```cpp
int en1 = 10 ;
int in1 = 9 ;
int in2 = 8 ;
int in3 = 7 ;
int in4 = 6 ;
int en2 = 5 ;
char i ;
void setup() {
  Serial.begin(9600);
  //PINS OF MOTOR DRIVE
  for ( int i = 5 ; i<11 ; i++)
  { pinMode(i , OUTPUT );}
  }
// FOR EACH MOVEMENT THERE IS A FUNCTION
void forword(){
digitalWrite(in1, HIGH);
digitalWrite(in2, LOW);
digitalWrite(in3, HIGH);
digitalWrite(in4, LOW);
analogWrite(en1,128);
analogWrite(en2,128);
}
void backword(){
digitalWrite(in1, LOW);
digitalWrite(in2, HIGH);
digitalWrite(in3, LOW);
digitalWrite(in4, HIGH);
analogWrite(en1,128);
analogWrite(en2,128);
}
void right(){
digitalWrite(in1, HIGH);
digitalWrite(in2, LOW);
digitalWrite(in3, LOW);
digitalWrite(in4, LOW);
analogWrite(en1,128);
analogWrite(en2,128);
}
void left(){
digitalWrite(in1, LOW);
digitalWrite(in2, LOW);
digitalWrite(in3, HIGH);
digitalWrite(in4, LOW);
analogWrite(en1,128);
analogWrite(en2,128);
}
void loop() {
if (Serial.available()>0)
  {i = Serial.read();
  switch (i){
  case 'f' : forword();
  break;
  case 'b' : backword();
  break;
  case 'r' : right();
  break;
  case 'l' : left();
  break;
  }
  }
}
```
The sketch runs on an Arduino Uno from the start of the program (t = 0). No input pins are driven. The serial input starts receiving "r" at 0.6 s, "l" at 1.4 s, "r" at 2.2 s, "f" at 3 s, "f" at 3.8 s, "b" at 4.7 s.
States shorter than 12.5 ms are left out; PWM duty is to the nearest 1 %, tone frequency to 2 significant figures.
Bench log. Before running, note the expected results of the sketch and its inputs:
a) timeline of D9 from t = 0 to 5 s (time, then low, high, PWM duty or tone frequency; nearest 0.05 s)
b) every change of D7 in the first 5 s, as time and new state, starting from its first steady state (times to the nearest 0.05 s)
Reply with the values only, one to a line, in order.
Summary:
0 s low; 0.6 s high; 1.4 s low; 2.2 s high; 4.7 s low
0 s low; 1.4 s high; 2.2 s low; 3 s high; 4.7 s low
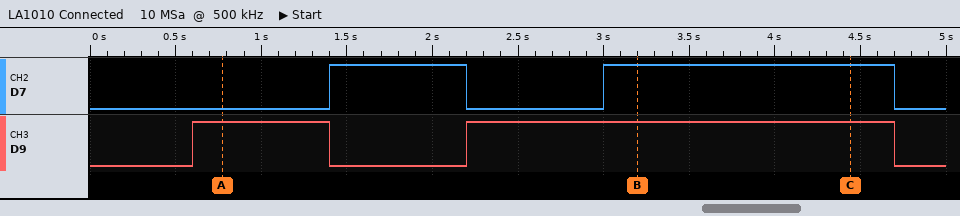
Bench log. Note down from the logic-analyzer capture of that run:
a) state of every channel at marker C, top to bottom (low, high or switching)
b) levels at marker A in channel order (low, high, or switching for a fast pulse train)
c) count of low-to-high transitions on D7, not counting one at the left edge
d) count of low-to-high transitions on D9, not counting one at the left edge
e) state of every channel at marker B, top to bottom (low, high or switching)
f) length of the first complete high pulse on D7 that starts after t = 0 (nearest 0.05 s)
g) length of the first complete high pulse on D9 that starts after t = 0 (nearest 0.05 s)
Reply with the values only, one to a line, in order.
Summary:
D7 high, D9 high
D7 low, D9 high
2
2
D7 high, D9 high
0.80 s
0.80 s
